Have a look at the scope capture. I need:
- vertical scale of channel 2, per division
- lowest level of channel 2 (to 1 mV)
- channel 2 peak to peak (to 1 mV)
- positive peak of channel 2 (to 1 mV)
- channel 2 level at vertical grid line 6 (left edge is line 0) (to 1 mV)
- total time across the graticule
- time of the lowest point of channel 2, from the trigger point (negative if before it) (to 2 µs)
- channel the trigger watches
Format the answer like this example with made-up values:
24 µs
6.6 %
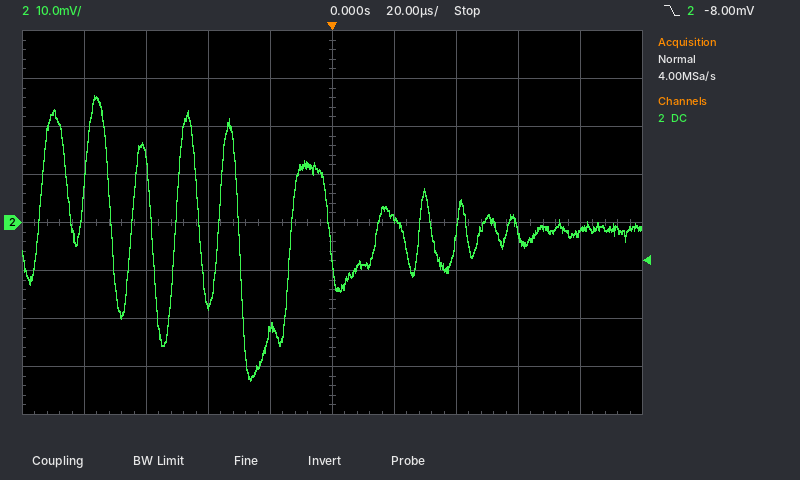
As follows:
10 mV
-33 mV
59 mV
26 mV
1 mV
200 µs
-26 µs
channel 2
